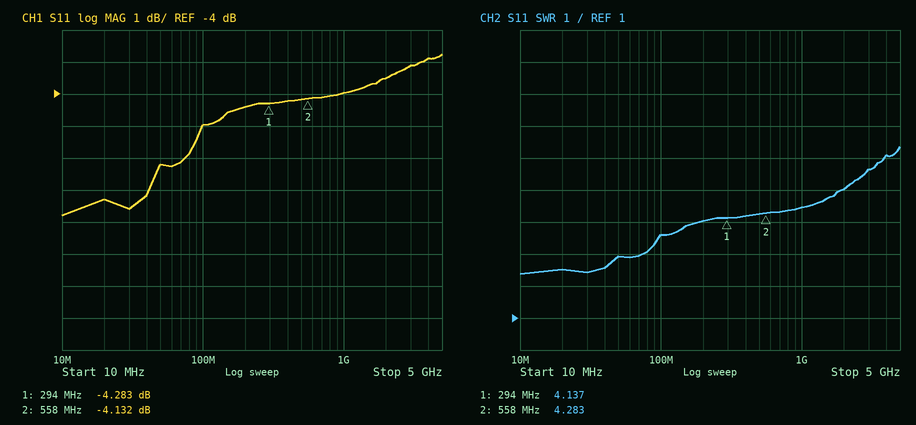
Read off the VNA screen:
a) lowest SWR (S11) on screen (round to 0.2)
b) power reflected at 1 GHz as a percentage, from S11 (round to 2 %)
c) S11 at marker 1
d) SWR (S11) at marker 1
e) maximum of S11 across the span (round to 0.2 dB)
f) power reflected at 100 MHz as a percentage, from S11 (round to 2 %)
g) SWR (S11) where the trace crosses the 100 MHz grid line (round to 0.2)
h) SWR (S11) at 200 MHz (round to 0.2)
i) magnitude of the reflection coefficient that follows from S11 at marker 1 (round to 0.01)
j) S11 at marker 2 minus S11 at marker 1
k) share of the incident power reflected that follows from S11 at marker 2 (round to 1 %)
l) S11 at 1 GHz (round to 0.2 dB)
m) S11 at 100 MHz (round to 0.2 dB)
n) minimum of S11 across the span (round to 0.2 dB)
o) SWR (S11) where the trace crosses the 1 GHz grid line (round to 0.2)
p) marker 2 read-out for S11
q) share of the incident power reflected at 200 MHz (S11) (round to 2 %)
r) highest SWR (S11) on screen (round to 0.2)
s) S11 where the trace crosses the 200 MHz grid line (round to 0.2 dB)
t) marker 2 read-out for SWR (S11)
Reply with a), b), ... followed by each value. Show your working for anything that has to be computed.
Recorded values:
a) 2.4
b) 10^(-4/10) ≈ 40 %
c) -4.283 dB
d) 4.137
e) -2.8 dB
f) 10^(-5/10) ≈ 32 %
g) 3.6
h) 4.0
i) 10^(-4.283/20) ≈ 0.61
j) -4.132 − (-4.283) = 0.151 dB
k) 10^(-4.132/10) ≈ 39 %
l) -4.0 dB
m) -5.0 dB
n) -7.8 dB
o) 4.4
p) -4.132 dB
q) 10^(-4.4/10) ≈ 36 %
r) 6.4
s) -4.4 dB
t) 4.283
